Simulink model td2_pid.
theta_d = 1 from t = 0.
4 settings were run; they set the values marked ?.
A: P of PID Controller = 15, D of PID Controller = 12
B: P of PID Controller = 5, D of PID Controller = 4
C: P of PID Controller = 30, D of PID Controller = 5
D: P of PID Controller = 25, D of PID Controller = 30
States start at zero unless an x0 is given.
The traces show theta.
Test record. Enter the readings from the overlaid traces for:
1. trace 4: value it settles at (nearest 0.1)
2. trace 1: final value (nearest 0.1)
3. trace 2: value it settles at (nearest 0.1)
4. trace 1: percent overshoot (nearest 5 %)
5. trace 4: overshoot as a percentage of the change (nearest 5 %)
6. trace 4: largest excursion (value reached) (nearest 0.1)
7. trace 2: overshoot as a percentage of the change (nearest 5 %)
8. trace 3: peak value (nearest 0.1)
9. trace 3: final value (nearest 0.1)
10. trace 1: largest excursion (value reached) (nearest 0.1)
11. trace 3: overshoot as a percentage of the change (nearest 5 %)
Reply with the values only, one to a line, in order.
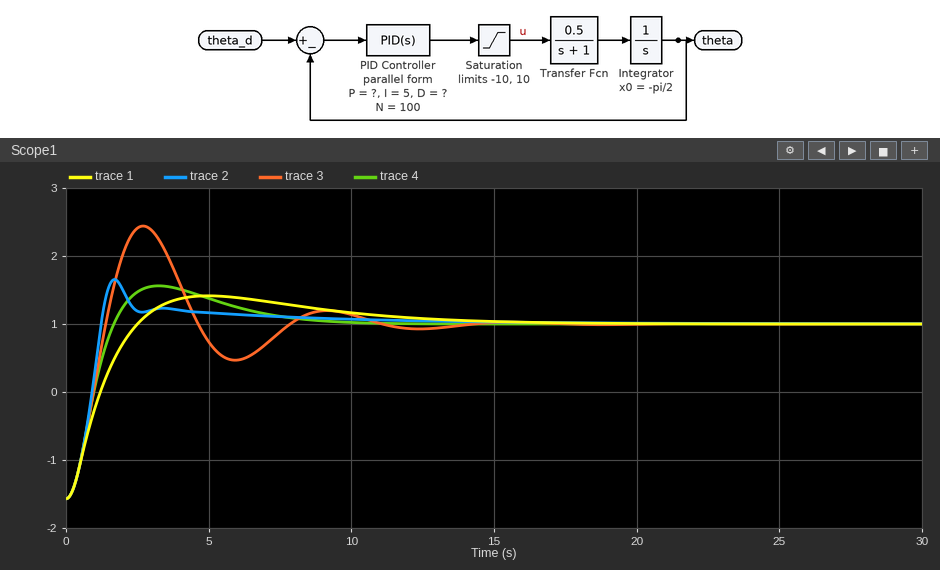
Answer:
1.0
1.0
1.0
15 %
20 %
1.6
25 %
2.4
1.0
1.4
55 %
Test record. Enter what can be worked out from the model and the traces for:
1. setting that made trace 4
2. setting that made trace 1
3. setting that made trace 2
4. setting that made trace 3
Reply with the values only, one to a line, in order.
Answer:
A
D
C
B
